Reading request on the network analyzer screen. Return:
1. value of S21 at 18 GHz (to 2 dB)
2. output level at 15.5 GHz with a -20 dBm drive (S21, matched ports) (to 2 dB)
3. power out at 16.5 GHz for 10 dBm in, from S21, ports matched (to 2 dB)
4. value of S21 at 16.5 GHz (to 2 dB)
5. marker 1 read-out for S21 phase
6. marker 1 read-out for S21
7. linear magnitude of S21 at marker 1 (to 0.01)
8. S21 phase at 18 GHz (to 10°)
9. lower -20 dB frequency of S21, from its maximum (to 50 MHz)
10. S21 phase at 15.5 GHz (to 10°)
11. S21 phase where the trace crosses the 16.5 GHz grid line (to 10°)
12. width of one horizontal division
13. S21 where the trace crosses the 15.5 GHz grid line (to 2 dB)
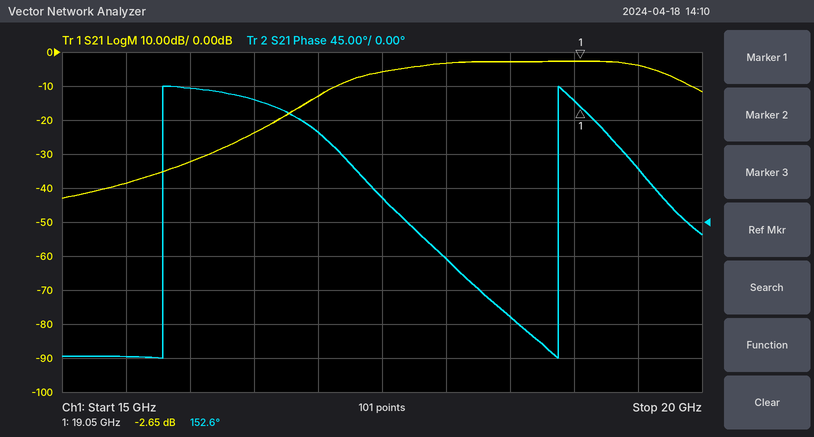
-4 dB
-58 dBm
-14 dBm
-24 dB
152.6°
-2.65 dB
0.74
-50°
16.55 GHz
-180°
160°
500 MHz
-38 dB
